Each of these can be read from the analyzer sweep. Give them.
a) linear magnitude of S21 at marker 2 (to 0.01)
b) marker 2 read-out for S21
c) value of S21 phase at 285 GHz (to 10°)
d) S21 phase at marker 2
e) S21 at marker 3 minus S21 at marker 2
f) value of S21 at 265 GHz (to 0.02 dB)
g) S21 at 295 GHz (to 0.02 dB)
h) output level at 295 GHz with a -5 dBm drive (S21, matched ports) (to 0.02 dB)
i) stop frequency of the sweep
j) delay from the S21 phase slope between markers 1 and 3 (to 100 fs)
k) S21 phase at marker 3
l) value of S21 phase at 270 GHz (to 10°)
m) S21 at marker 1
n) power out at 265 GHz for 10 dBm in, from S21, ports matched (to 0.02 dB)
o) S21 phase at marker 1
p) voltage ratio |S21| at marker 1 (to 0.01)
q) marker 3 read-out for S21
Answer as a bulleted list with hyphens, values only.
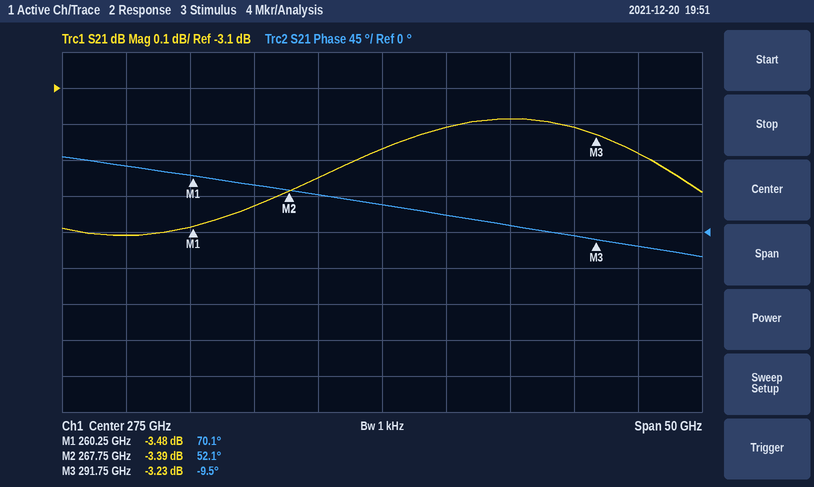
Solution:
- 0.68
- -3.39 dB
- 10°
- 52.1°
- 0.16 dB
- -3.42 dB
- -3.28 dB
- -8.28 dBm
- 300 GHz
- 7.0 ps
- -9.5°
- 50°
- -3.48 dB
- 6.58 dBm
- 70.1°
- 0.67
- -3.23 dB
